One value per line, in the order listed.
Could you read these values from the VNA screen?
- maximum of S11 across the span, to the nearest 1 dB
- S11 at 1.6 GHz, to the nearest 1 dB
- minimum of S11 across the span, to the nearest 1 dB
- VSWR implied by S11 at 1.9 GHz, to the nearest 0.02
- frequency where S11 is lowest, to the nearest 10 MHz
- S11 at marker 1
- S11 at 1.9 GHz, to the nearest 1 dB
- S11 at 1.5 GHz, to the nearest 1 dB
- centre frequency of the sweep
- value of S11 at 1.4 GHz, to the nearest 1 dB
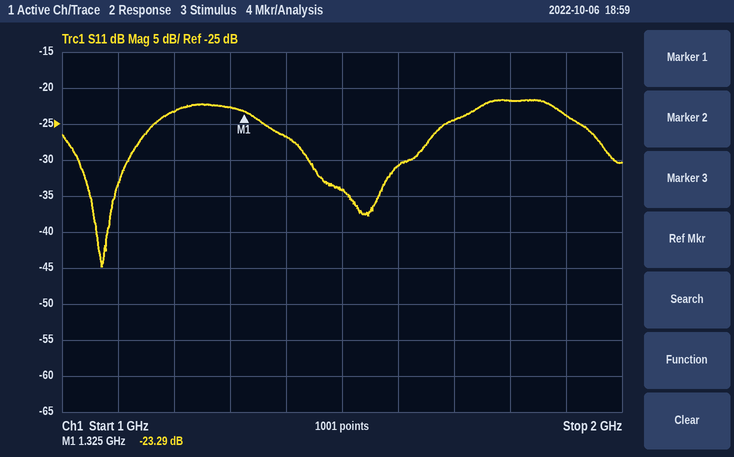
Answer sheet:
-22 dB
-31 dB
-45 dB
1.14
1.07 GHz
-23.29 dB
-24 dB
-34 dB
1.5 GHz
-27 dB
